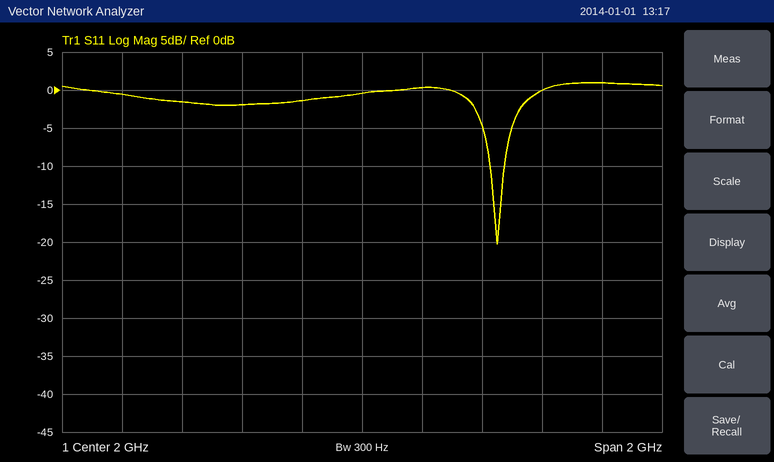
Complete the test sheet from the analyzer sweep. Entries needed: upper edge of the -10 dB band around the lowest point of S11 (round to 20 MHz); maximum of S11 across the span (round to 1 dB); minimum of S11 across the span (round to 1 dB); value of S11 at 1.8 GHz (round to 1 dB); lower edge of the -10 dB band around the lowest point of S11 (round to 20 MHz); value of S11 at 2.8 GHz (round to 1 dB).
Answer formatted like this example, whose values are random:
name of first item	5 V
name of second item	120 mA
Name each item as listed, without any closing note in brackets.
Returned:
upper edge of the -10 dB band around the lowest point of S11	2.48 GHz
maximum of S11 across the span	1 dB
minimum of S11 across the span	-20 dB
value of S11 at 1.8 GHz	-1 dB
lower edge of the -10 dB band around the lowest point of S11	2.42 GHz
value of S11 at 2.8 GHz	1 dB
